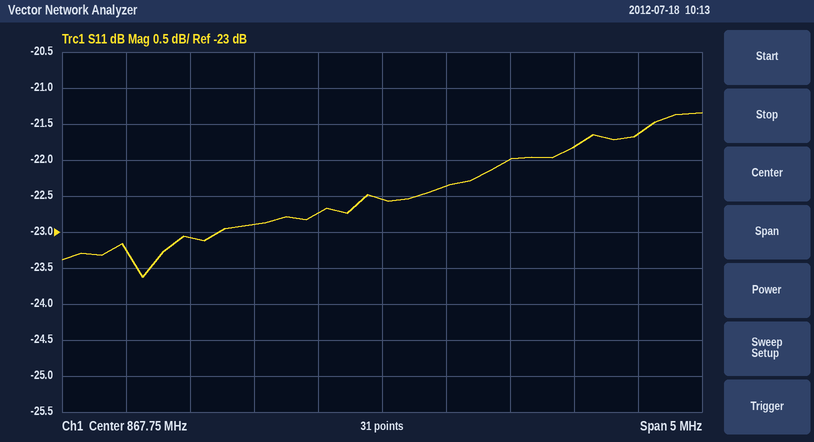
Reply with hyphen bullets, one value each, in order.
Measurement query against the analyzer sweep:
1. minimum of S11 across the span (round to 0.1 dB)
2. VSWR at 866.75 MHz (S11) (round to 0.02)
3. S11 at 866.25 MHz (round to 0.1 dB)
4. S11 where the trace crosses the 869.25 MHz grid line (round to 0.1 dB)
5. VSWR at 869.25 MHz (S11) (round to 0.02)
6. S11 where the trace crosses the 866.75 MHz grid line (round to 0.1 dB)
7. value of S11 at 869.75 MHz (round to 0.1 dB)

- -23.6 dB
- 1.16
- -23.1 dB
- -21.8 dB
- 1.18
- -22.9 dB
- -21.6 dB
